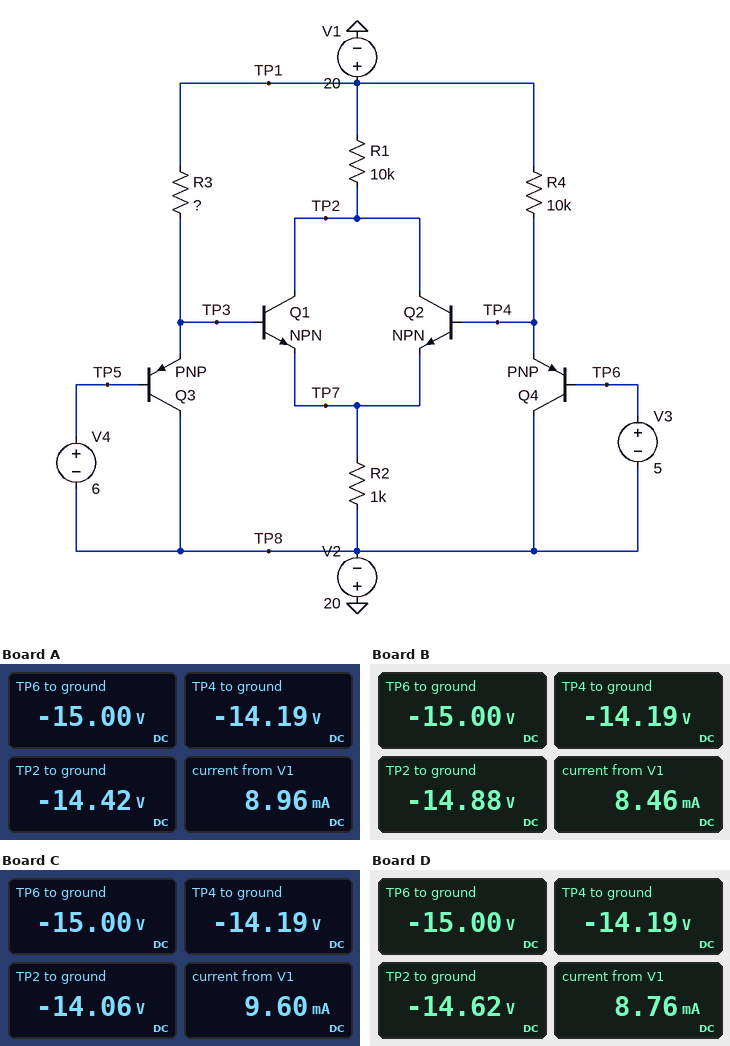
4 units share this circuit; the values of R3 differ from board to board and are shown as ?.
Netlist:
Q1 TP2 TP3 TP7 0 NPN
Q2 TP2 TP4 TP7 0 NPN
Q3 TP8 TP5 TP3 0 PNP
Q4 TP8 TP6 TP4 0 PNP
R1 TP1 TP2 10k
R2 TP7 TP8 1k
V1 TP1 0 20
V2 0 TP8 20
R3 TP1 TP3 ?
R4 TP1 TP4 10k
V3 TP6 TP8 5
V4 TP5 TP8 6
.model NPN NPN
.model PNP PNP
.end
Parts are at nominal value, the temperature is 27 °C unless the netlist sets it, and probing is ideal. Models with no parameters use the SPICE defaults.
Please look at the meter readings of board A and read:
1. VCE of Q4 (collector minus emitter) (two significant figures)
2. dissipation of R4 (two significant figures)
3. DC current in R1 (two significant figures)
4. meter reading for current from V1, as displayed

-5.8 V
120 mW
3.4 mA
8.96 mA
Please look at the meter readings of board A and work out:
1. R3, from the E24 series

16 kΩ
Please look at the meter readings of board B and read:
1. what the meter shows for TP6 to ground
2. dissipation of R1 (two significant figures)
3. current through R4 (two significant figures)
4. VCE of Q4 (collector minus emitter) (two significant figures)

-15.00 V
120 mW
3.4 mA
-5.8 V
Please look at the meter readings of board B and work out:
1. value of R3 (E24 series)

22 kΩ
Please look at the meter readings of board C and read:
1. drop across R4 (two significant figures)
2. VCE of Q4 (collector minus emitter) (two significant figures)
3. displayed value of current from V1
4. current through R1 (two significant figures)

34 V
-5.8 V
9.60 mA
3.4 mA
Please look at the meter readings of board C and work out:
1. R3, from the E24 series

12 kΩ
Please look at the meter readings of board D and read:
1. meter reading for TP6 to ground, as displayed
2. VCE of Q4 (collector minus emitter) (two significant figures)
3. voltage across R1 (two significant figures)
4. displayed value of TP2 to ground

-15.00 V
-5.8 V
35 V
-14.62 V
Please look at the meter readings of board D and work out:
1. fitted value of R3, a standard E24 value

18 kΩ
